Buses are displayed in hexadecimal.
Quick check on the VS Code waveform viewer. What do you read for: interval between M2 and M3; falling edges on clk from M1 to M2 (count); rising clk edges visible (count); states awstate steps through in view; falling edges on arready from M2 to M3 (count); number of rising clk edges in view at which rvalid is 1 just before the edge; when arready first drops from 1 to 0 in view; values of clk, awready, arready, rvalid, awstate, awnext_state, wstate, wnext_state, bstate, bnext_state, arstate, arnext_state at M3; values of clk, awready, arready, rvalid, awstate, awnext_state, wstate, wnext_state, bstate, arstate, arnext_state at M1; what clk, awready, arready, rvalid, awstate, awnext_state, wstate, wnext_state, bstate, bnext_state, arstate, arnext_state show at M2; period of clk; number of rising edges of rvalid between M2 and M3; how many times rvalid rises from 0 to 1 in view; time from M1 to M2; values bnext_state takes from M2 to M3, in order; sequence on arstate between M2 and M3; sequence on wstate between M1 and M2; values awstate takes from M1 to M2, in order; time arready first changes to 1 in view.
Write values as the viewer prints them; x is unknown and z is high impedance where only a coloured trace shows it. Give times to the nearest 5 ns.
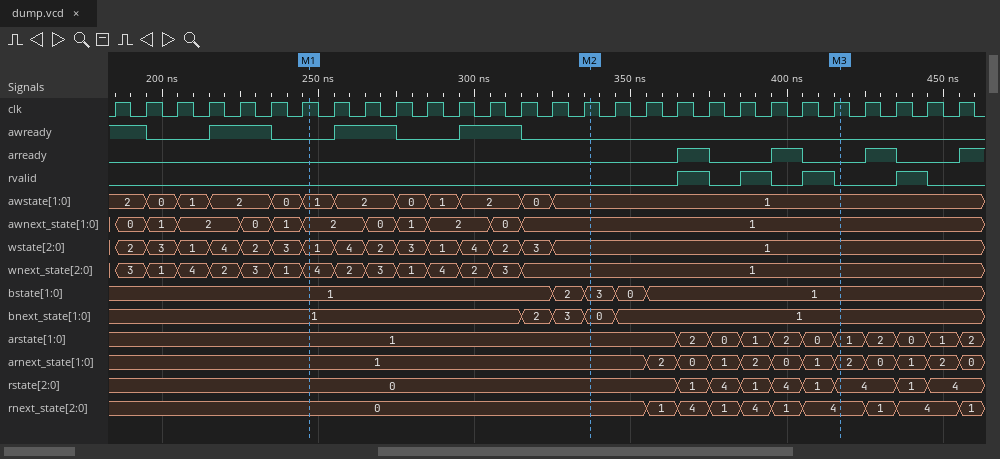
80 ns
9
28
2, 0, 1, 2, 0, 1, 2, 0, 1, 2, 0, 1
2
4
375 ns
clk=1, awready=0, arready=0, rvalid=0, awstate=1, awnext_state=1, wstate=1, wnext_state=1, bstate=1, bnext_state=1, arstate=1, arnext_state=2
clk=1, awready=0, arready=0, rvalid=0, awstate=1, awnext_state=2, wstate=1, wnext_state=4, bstate=1, arstate=1, arnext_state=1
clk=1, awready=0, arready=0, rvalid=0, awstate=1, awnext_state=1, wstate=1, wnext_state=1, bstate=3, bnext_state=0, arstate=1, arnext_state=1
10 ns
3
4
90 ns
0, 1
1, 2, 0, 1, 2, 0, 1
1, 4, 2, 3, 1, 4, 2, 3, 1
1, 2, 0, 1, 2, 0, 1
365 ns
